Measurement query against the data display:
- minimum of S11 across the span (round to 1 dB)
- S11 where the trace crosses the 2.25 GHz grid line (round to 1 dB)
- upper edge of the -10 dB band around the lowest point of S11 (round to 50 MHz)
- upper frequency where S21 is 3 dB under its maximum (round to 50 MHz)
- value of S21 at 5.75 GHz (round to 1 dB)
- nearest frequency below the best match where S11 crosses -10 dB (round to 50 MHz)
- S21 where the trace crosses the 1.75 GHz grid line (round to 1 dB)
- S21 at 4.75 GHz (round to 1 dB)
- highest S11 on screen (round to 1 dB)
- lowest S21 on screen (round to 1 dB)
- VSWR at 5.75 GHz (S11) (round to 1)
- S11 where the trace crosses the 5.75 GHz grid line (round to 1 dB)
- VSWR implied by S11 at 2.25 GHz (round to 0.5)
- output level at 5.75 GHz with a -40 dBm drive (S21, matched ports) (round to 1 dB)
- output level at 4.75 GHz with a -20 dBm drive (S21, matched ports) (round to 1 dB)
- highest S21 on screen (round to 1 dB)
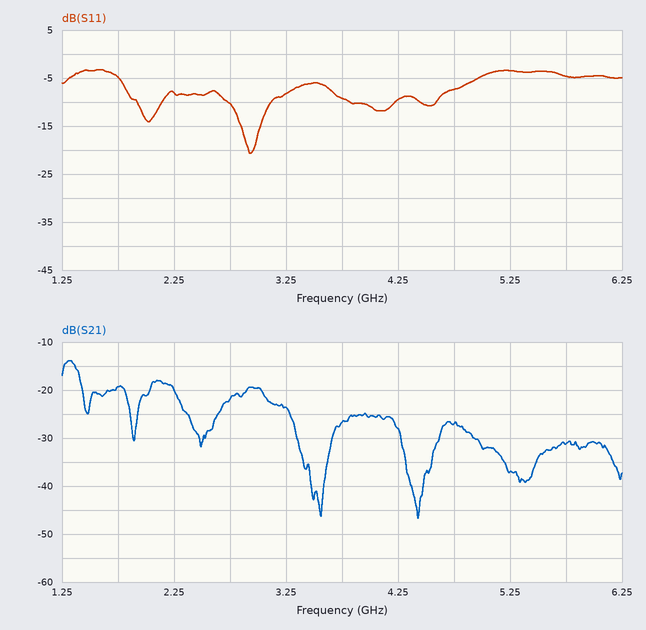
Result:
-21 dB
-8 dB
3.10 GHz
1.40 GHz
-31 dB
2.75 GHz
-19 dB
-27 dB
-3 dB
-47 dB
4
-5 dB
2.5
-71 dBm
-47 dBm
-14 dB
